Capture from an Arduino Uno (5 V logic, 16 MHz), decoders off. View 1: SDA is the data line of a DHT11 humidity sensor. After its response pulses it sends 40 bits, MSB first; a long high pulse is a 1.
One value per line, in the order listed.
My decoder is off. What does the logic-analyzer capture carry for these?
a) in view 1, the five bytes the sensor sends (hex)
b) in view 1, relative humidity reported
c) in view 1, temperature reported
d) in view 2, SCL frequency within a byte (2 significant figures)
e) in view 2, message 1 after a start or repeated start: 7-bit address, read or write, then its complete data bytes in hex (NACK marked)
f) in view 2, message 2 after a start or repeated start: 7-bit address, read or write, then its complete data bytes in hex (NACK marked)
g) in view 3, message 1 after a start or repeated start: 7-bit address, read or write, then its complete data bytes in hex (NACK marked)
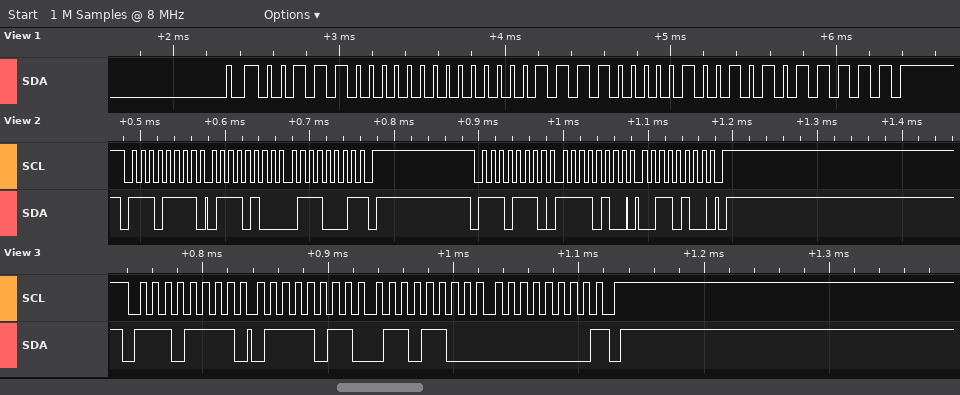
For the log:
38 00 1E 09 5F
56 %
30.9 °C
100 kHz
0x77 read: 74 71 NACK
0x77 write: F4 34
0x77 read: 7B 6C 00 NACK
